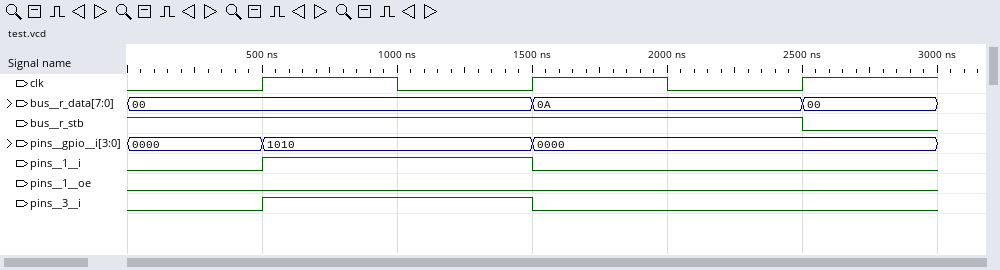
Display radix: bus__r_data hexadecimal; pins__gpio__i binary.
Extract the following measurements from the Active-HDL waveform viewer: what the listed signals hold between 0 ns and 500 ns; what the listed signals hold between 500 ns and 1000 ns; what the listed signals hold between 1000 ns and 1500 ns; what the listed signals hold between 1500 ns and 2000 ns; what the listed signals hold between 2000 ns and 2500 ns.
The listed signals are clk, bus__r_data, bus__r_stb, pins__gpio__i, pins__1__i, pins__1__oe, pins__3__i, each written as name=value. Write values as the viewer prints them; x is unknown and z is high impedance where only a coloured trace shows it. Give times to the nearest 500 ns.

clk=0, bus__r_data=00, bus__r_stb=1, pins__gpio__i=0000, pins__1__i=0, pins__1__oe=0, pins__3__i=0
clk=1, bus__r_data=00, bus__r_stb=1, pins__gpio__i=1010, pins__1__i=1, pins__1__oe=0, pins__3__i=1
clk=0, bus__r_data=00, bus__r_stb=1, pins__gpio__i=1010, pins__1__i=1, pins__1__oe=0, pins__3__i=1
clk=1, bus__r_data=0A, bus__r_stb=1, pins__gpio__i=0000, pins__1__i=0, pins__1__oe=0, pins__3__i=0
clk=0, bus__r_data=0A, bus__r_stb=1, pins__gpio__i=0000, pins__1__i=0, pins__1__oe=0, pins__3__i=0
